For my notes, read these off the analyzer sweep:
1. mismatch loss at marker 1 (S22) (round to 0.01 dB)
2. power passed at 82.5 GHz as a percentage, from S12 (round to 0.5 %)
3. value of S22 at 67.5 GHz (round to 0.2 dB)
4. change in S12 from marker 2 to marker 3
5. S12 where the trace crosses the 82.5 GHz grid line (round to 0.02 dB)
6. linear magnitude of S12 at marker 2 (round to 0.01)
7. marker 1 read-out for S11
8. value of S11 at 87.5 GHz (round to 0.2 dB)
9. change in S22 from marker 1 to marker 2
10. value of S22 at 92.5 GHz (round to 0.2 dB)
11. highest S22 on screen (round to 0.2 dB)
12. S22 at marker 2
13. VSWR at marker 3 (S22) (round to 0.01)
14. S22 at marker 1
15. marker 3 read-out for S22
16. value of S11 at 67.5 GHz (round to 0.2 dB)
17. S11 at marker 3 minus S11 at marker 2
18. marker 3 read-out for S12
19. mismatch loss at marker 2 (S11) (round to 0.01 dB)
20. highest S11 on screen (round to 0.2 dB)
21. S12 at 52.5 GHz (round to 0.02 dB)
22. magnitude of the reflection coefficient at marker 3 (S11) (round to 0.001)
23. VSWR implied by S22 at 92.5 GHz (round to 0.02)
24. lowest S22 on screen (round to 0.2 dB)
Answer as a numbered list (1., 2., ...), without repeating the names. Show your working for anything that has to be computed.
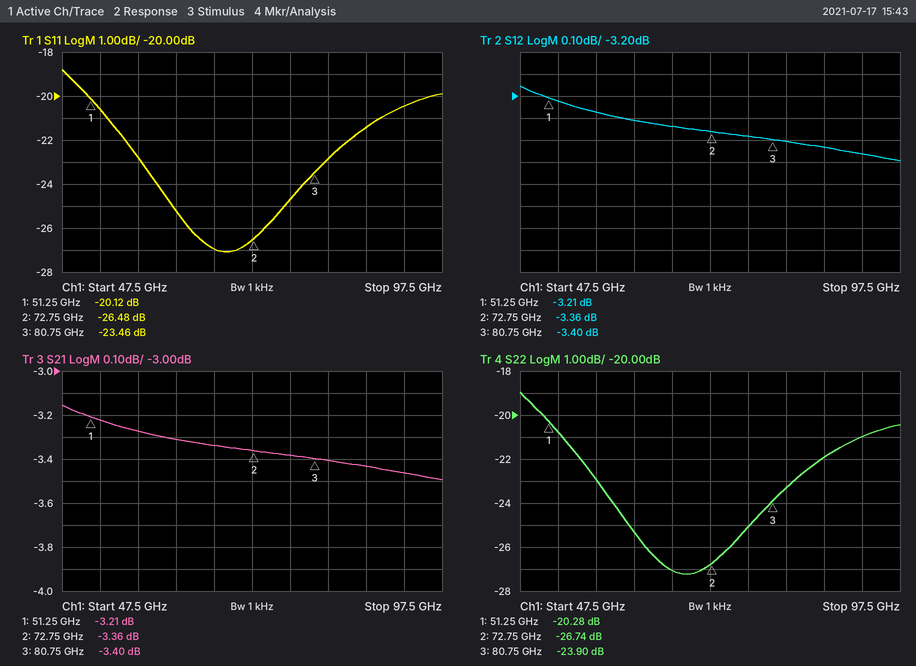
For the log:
1. −10 log10(1 − 10^(-20.28/10)) ≈ 0.04 dB
2. 10^(-3.4/10) ≈ 45.7 %, so 45.5 % to the nearest 0.5 %
3. -27.0 dB
4. -3.4 − (-3.36) = -0.04 dB
5. -3.40 dB
6. 10^(-3.36/20) ≈ 0.68
7. -20.12 dB
8. -21.4 dB
9. -26.74 − (-20.28) = -6.46 dB
10. -21.0 dB
11. -19.0 dB
12. -26.74 dB
13. (1 + 0.0638)/(1 − 0.0638) ≈ 1.14
14. -20.28 dB
15. -23.90 dB
16. -27.0 dB
17. -23.46 − (-26.48) = 3.02 dB
18. -3.40 dB
19. −10 log10(1 − 10^(-26.48/10)) ≈ 0.01 dB
20. -18.8 dB
21. -3.22 dB
22. 10^(-23.46/20) ≈ 0.067
23. |Γ| = 10^(-21/20) = 0.0891; VSWR = (1 + 0.0891)/(1 − 0.0891) ≈ 1.20
24. -27.2 dB
